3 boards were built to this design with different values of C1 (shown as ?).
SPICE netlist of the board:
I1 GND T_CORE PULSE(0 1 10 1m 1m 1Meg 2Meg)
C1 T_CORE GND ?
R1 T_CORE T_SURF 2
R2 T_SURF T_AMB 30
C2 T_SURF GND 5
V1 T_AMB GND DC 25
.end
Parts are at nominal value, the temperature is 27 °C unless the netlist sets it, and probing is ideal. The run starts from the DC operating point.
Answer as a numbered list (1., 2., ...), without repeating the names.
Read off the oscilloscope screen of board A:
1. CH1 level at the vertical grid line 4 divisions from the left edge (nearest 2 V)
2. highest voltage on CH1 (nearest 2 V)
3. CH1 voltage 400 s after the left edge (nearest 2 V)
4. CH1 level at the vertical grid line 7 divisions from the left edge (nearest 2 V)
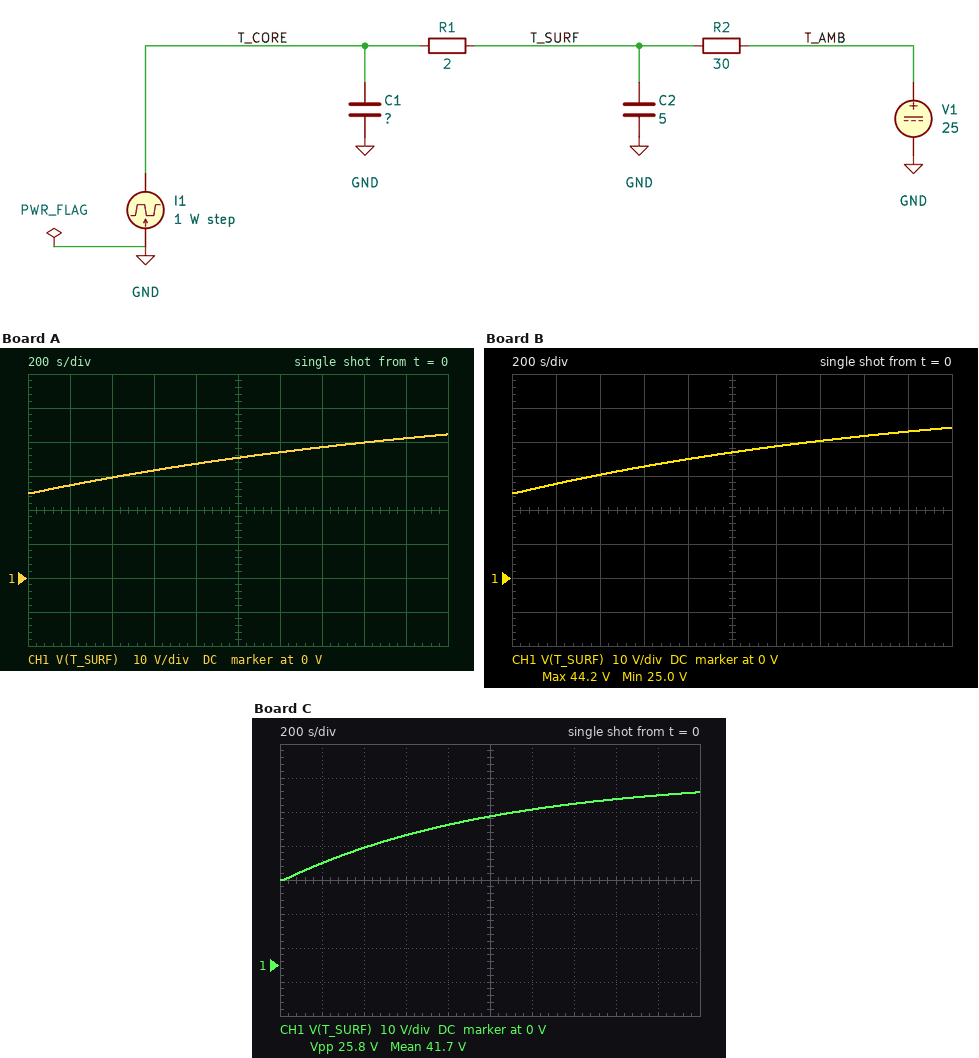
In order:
1. 34 V
2. 42 V
3. 30 V
4. 38 V
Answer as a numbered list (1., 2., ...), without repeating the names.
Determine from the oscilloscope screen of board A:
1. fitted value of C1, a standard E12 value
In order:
1. 68 F
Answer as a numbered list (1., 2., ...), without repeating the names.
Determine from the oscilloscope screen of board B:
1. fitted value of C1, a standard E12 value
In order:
1. 56 F
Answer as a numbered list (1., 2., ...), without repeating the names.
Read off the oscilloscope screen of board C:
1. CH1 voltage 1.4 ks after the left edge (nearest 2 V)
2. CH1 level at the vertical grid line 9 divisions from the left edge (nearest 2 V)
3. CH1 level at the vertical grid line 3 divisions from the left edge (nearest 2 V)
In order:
1. 48 V
2. 50 V
3. 38 V
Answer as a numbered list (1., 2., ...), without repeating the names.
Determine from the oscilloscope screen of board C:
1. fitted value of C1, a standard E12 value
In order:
1. 27 F
